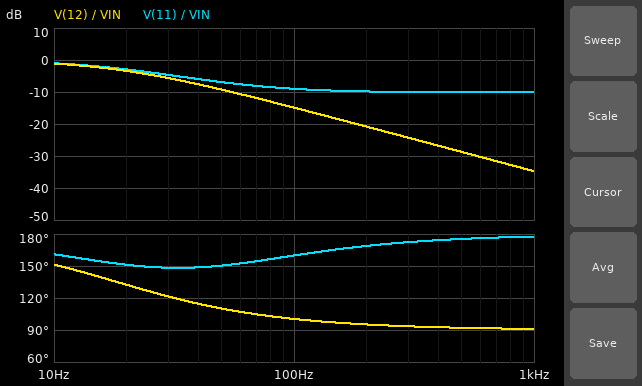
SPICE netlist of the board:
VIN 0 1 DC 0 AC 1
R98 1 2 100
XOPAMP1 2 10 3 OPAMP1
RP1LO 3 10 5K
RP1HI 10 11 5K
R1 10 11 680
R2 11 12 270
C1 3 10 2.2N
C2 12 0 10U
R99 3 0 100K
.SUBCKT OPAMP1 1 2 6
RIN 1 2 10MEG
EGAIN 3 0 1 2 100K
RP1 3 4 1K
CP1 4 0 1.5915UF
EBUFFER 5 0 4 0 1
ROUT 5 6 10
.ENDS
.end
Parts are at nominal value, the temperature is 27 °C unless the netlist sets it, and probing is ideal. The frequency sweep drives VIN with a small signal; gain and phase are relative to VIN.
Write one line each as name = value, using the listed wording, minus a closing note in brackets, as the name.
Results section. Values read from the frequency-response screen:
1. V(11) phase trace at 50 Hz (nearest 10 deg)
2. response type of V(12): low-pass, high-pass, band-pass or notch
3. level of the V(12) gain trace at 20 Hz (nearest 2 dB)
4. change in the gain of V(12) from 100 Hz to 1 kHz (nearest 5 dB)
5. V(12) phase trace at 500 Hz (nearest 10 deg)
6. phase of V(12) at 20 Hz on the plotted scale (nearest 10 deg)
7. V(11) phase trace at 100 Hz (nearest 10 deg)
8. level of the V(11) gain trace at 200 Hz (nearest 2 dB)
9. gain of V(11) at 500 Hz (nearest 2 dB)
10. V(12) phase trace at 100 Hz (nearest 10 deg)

V(11) phase trace at 50 Hz = 150 deg
response type of V(12): low-pass, high-pass, band-pass or notch = low-pass
level of the V(12) gain trace at 20 Hz = -4 dB
change in the gain of V(12) from 100 Hz to 1 kHz = -20 dB
V(12) phase trace at 500 Hz = 90 deg
phase of V(12) at 20 Hz on the plotted scale = 130 deg
V(11) phase trace at 100 Hz = 160 deg
level of the V(11) gain trace at 200 Hz = -10 dB
gain of V(11) at 500 Hz = -10 dB
V(12) phase trace at 100 Hz = 100 deg
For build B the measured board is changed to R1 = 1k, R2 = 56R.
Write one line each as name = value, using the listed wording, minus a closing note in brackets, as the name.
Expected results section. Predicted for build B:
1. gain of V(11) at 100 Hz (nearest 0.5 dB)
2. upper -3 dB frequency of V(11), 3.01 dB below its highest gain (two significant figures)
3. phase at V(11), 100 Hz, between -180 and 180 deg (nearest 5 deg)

gain of V(11) at 100 Hz = -14.5 dB
upper -3 dB frequency of V(11), 3.01 dB below its highest gain = 18 Hz
phase at V(11), 100 Hz, between -180 and 180 deg = 120 deg
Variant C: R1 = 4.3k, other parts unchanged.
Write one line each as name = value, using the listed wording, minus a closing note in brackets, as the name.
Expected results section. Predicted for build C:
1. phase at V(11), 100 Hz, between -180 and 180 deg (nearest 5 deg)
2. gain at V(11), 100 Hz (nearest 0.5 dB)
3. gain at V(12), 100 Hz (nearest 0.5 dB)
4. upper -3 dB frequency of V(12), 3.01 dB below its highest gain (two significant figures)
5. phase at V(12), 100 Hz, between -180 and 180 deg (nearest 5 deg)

phase at V(11), 100 Hz, between -180 and 180 deg = 155 deg
gain at V(11), 100 Hz = -18.5 dB
gain at V(12), 100 Hz = -24.0 dB
upper -3 dB frequency of V(12), 3.01 dB below its highest gain = 6.2 Hz
phase at V(12), 100 Hz, between -180 and 180 deg = 95 deg
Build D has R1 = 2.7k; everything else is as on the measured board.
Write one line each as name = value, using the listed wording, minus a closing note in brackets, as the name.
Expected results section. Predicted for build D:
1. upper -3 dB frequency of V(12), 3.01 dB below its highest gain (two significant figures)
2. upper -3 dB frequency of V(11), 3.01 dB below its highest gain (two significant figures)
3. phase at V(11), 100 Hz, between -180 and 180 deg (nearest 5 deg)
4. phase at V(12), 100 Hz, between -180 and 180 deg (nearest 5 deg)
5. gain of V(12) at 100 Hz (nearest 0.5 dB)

upper -3 dB frequency of V(12), 3.01 dB below its highest gain = 7.9 Hz
upper -3 dB frequency of V(11), 3.01 dB below its highest gain = 8.0 Hz
phase at V(11), 100 Hz, between -180 and 180 deg = 155 deg
phase at V(12), 100 Hz, between -180 and 180 deg = 95 deg
gain of V(12) at 100 Hz = -22.0 dB
